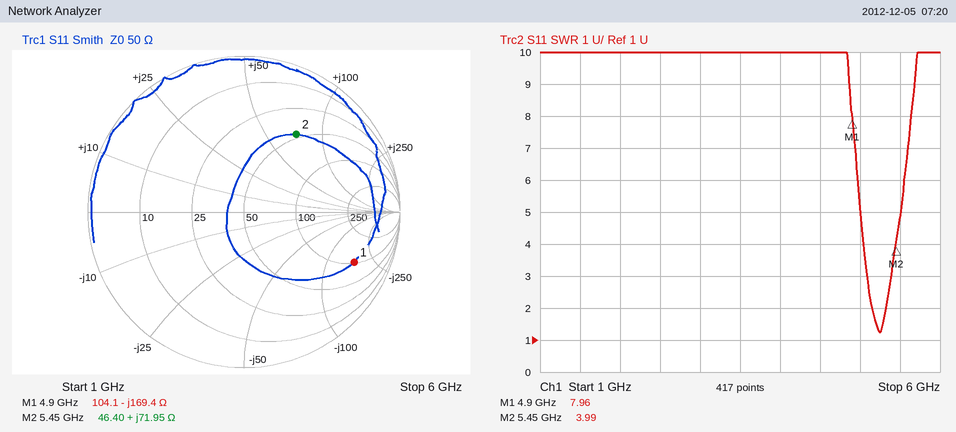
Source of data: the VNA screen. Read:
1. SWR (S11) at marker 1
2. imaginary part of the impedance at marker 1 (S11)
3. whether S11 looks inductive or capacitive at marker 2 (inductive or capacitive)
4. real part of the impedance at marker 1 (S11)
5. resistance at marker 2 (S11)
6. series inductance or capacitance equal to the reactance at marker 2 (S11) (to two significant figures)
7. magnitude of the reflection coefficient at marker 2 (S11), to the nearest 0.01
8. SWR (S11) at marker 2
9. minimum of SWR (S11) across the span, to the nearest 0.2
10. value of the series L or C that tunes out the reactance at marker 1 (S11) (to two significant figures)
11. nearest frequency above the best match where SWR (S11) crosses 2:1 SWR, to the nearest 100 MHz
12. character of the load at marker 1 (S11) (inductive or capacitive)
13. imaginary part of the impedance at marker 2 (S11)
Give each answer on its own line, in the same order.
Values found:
7.96
-169.4 Ω
inductive
104.1 Ω
46.40 Ω
2.1 nH
0.60
3.99
1.2
5.5 nH
5.3 GHz
capacitive
+71.95 Ω
